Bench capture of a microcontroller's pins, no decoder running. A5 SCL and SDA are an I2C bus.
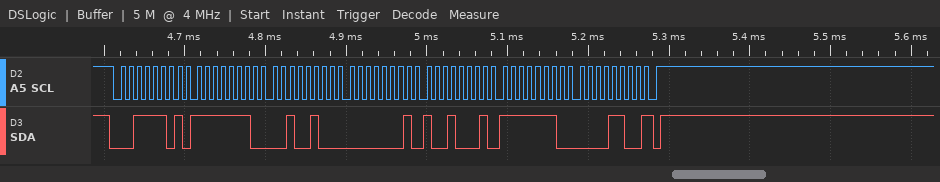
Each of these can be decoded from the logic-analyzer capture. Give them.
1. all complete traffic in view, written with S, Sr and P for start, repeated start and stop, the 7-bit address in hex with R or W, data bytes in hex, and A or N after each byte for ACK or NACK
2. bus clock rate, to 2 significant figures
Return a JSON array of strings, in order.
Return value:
["S 1ER A FE A 24 A 01 A 91 A FE A 0C N P", "100 kHz"]
